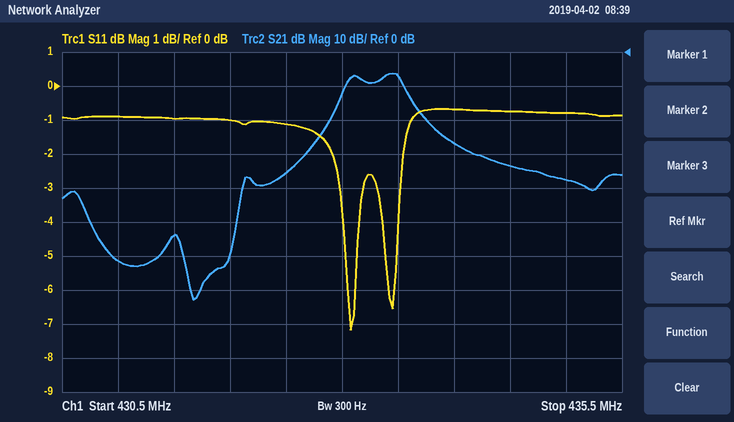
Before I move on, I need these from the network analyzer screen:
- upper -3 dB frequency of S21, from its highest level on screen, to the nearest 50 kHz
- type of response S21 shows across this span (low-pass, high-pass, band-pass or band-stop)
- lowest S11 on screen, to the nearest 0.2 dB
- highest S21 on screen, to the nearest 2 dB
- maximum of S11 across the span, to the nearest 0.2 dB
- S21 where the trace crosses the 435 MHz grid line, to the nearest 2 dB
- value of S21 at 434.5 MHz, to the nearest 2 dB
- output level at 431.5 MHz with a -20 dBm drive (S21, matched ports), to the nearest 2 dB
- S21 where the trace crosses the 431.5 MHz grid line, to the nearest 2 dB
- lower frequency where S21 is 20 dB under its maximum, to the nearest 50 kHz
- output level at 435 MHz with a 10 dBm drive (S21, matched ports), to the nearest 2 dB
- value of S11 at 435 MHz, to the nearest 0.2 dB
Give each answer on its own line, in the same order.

433.55 MHz
band-pass
-7.2 dB
-6 dB
-0.6 dB
-38 dB
-34 dB
-74 dBm
-54 dB
432.75 MHz
-28 dBm
-0.8 dB
